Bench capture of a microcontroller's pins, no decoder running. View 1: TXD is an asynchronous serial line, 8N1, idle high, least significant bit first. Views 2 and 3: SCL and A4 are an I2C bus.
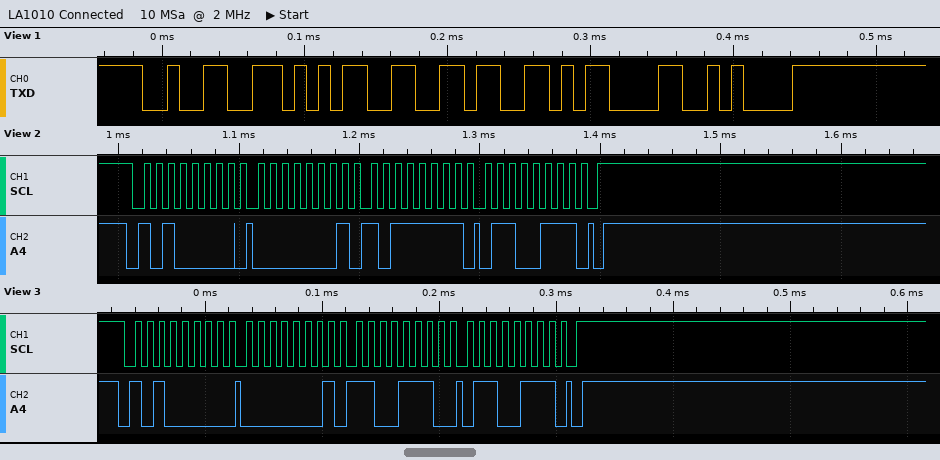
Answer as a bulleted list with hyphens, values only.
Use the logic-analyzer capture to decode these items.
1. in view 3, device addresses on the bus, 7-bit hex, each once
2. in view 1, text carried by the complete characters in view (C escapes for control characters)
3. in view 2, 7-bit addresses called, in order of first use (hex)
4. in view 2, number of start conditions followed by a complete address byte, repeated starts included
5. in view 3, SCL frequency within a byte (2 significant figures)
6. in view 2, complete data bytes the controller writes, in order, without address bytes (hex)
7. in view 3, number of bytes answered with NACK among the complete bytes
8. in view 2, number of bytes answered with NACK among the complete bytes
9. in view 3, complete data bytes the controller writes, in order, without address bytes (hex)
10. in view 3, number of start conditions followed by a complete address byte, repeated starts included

- 0x50
- "256\r\n"
- 0x50
- 1
- 100 kHz
- 01 BF 67
- 0
- 0
- 01 CE 67
- 1
